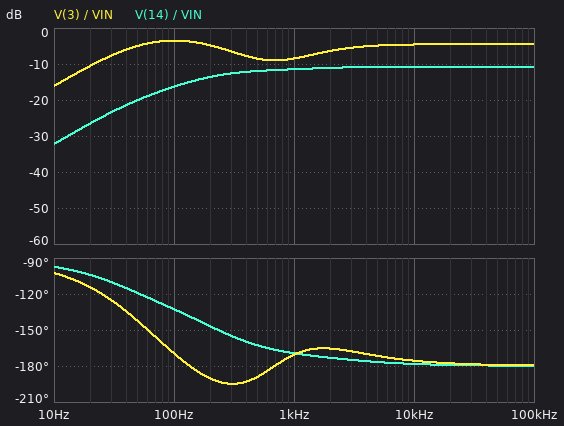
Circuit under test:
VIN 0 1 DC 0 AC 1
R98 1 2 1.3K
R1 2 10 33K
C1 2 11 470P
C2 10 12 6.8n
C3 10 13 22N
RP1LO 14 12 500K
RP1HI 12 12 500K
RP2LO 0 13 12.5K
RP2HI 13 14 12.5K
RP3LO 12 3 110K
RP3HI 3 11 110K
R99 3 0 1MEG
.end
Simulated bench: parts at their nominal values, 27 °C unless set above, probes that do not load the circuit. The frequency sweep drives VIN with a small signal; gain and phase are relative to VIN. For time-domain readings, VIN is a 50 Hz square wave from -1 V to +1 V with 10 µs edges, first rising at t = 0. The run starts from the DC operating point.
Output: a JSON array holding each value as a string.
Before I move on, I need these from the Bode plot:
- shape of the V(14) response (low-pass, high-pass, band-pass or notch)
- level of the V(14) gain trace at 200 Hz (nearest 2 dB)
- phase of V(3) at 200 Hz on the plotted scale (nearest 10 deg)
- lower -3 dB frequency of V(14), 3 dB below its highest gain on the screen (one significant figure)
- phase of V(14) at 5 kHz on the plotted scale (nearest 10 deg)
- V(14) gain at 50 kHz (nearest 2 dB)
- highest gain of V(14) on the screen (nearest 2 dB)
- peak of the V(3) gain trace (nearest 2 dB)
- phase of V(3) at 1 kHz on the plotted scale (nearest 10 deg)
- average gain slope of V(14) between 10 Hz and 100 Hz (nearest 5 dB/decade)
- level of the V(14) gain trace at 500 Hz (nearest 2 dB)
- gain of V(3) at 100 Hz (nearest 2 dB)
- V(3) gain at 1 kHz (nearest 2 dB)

["high-pass", "-14 dB", "-190 deg", "200 Hz", "-180 deg", "-10 dB", "-10 dB", "-4 dB", "-170 deg", "15 dB/decade", "-12 dB", "-4 dB", "-8 dB"]
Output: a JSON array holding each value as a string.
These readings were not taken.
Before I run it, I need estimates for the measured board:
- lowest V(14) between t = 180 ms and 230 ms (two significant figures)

["-570 mV"]
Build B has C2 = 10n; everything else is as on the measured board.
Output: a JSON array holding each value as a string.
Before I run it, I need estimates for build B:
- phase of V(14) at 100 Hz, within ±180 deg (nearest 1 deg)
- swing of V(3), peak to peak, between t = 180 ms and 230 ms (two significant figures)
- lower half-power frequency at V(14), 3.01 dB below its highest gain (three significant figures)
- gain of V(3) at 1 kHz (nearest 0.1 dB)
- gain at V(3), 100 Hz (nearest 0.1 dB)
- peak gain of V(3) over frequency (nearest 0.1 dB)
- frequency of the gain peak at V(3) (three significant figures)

["-134 deg", "2.0 V", "198 Hz", "-8.7 dB", "-3.1 dB", "-3.0 dB", "83.0 Hz"]
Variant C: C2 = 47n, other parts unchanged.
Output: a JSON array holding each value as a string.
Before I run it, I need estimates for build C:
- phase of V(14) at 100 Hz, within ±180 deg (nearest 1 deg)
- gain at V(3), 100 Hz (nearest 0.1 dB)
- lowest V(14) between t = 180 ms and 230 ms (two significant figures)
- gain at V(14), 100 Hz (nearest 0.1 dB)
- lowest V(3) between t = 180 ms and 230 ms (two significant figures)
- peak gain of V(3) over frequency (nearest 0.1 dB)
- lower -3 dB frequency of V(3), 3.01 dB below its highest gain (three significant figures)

["-136 deg", "-2.9 dB", "-540 mV", "-17.0 dB", "-870 mV", "-2.0 dB", "7.82 Hz"]
